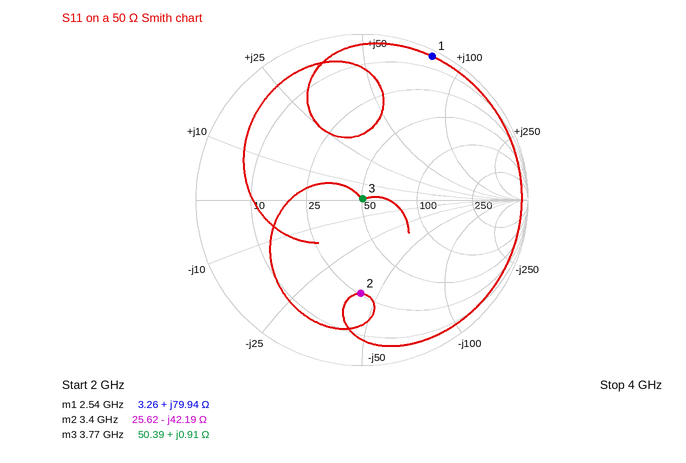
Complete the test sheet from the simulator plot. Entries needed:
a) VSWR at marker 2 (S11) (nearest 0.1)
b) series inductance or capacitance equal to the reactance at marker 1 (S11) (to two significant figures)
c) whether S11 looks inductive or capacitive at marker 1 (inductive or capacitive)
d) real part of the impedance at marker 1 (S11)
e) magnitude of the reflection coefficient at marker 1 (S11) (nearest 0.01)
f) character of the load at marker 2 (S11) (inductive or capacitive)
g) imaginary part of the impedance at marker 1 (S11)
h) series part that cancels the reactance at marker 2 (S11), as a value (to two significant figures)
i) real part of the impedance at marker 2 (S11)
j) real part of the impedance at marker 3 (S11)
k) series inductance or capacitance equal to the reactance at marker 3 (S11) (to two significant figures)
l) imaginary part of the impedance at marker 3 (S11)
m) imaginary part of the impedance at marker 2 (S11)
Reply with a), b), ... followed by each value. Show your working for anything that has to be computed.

a) 3.6
b) L = 79.94 Ω/(2π × 2.54 GHz) ≈ 5.0 nH
c) inductive
d) 3.26 Ω
e) 0.96
f) capacitive
g) +79.94 Ω
h) L = 42.19 Ω/(2π × 3.4 GHz) ≈ 2.0 nH
i) 25.62 Ω
j) 50.39 Ω
k) L = 0.91 Ω/(2π × 3.77 GHz) ≈ 38 pH
l) +0.91 Ω
m) -42.19 Ω
